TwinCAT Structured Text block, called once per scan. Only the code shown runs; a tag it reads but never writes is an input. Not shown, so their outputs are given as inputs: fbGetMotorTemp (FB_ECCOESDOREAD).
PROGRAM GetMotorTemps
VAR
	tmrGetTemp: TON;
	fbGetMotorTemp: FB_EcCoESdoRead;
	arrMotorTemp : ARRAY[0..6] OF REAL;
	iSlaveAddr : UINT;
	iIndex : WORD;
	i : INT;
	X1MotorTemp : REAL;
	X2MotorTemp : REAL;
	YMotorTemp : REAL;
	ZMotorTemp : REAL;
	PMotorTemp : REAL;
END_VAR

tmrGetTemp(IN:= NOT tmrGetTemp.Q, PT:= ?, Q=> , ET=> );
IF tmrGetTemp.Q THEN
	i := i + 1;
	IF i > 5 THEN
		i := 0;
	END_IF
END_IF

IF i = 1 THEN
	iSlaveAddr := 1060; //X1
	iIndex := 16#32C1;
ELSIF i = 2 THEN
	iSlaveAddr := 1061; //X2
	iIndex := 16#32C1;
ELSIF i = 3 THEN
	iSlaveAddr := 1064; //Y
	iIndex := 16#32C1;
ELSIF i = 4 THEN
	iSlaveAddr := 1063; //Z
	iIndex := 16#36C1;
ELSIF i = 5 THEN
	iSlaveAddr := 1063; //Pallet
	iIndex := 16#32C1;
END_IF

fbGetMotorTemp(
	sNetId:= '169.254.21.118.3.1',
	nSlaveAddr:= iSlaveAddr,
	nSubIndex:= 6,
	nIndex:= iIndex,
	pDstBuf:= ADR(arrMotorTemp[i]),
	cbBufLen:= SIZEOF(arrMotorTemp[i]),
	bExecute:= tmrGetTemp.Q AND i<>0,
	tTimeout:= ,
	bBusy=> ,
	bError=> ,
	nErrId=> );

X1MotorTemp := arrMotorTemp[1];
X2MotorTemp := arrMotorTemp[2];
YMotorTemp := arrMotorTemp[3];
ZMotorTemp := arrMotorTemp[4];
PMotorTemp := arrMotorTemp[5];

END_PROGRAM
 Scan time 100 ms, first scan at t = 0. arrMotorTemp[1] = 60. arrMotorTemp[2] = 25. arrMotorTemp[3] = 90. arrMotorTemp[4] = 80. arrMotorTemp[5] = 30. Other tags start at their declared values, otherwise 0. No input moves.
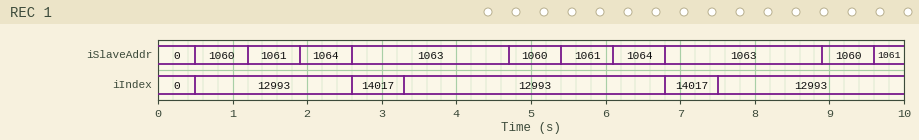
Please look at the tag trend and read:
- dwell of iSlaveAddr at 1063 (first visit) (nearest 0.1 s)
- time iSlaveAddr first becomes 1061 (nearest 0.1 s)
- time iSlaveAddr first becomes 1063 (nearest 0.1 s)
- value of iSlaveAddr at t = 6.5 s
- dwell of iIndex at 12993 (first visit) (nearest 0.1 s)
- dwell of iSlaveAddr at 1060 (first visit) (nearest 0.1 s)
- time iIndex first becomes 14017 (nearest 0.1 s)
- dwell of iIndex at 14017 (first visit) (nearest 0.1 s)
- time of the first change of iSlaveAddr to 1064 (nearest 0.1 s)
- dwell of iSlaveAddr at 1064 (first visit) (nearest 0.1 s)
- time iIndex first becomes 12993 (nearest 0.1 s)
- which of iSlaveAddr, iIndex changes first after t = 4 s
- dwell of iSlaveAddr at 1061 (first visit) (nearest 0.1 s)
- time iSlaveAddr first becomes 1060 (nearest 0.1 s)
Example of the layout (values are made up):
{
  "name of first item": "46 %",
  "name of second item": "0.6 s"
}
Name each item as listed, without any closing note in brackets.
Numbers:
{
  "dwell of iSlaveAddr at 1063 (first visit)": "2.1 s",
  "time iSlaveAddr first becomes 1061": "1.2 s",
  "time iSlaveAddr first becomes 1063": "2.6 s",
  "value of iSlaveAddr at t = 6.5 s": "1064",
  "dwell of iIndex at 12993 (first visit)": "2.1 s",
  "dwell of iSlaveAddr at 1060 (first visit)": "0.7 s",
  "time iIndex first becomes 14017": "2.6 s",
  "dwell of iIndex at 14017 (first visit)": "0.7 s",
  "time of the first change of iSlaveAddr to 1064": "1.9 s",
  "dwell of iSlaveAddr at 1064 (first visit)": "0.7 s",
  "time iIndex first becomes 12993": "0.5 s",
  "which of iSlaveAddr, iIndex changes first after t = 4 s": "iSlaveAddr",
  "dwell of iSlaveAddr at 1061 (first visit)": "0.7 s",
  "time iSlaveAddr first becomes 1060": "0.5 s"
}
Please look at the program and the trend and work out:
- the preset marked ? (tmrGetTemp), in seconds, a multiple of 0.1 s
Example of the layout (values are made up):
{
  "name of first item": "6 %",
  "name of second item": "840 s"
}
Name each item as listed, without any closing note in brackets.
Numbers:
{
  "the preset marked ? (tmrGetTemp), in seconds, a multiple of 0.1 s": "0.5 s"
}
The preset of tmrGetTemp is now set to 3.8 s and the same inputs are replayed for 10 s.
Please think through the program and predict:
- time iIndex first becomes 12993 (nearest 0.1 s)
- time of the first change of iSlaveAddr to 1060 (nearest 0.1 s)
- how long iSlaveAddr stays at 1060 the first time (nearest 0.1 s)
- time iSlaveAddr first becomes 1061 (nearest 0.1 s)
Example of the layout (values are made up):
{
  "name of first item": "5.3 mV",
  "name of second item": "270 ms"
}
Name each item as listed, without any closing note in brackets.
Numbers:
{
  "time iIndex first becomes 12993": "3.8 s",
  "time of the first change of iSlaveAddr to 1060": "3.8 s",
  "how long iSlaveAddr stays at 1060 the first time": "4.0 s",
  "time iSlaveAddr first becomes 1061": "7.8 s"
}
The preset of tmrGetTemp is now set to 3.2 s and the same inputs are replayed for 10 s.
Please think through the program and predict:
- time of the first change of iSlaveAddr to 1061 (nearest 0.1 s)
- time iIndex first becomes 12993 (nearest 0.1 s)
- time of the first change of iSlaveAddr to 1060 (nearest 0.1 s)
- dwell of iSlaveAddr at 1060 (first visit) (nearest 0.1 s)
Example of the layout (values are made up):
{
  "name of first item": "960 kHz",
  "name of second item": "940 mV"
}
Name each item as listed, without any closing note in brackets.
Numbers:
{
  "time of the first change of iSlaveAddr to 1061": "6.6 s",
  "time iIndex first becomes 12993": "3.2 s",
  "time of the first change of iSlaveAddr to 1060": "3.2 s",
  "dwell of iSlaveAddr at 1060 (first visit)": "3.4 s"
}
